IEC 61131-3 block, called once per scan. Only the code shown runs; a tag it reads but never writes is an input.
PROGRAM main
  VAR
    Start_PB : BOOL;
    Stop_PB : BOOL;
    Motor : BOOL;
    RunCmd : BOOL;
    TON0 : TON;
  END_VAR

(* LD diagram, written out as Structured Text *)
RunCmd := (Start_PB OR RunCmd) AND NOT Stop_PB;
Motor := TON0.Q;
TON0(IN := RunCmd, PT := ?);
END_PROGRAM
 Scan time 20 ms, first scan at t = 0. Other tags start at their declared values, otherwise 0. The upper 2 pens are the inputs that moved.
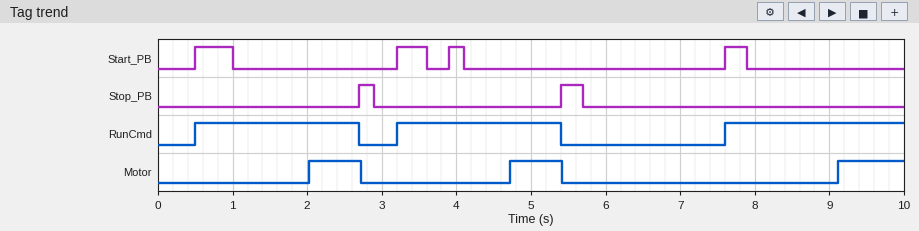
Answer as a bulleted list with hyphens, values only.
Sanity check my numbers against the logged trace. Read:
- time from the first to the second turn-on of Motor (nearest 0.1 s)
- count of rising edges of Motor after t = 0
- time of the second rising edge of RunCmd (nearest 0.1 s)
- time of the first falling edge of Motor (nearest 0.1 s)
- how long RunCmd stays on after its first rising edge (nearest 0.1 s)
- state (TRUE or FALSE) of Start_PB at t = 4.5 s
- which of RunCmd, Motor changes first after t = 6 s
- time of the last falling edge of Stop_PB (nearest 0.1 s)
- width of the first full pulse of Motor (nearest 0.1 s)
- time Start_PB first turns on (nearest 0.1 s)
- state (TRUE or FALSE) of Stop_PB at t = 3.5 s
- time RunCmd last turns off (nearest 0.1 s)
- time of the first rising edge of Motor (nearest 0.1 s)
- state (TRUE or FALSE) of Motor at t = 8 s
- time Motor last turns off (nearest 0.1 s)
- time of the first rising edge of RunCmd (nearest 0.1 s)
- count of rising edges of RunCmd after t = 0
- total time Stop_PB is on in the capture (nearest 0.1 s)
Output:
- 2.7 s
- 3
- 3.2 s
- 2.7 s
- 2.2 s
- FALSE
- RunCmd
- 5.7 s
- 0.7 s
- 0.5 s
- FALSE
- 5.4 s
- 2.0 s
- FALSE
- 5.4 s
- 0.5 s
- 3
- 0.5 s
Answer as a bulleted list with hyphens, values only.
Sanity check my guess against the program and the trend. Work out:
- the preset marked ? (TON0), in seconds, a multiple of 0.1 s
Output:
- 1.5 s
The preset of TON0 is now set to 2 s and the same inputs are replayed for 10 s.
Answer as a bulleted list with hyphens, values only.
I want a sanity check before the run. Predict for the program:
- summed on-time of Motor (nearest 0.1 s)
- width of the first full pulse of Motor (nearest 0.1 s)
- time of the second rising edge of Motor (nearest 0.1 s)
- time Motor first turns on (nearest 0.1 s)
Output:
- 0.8 s
- 0.2 s
- 5.2 s
- 2.5 s
